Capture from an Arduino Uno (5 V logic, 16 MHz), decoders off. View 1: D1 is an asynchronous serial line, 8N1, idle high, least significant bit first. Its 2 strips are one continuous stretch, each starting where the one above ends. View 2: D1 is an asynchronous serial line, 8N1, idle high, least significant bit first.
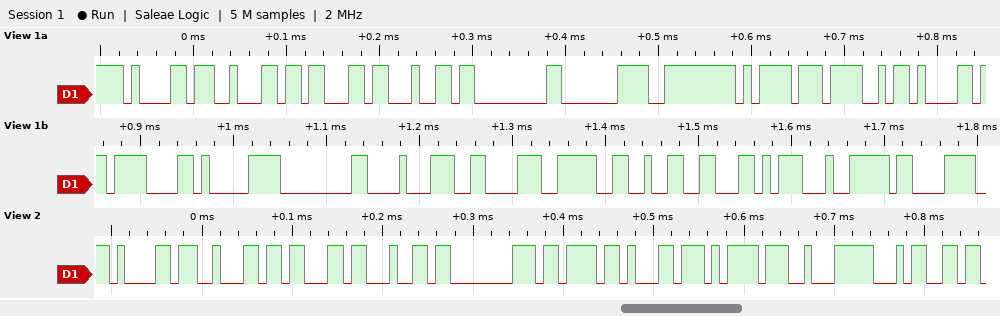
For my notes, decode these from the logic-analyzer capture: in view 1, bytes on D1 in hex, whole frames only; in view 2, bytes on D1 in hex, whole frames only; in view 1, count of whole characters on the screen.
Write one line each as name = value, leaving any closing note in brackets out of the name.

in view 1, bytes on D1 in hex, whole frames only = 0x61 0x62 0x63 0x64 0x00 0xC0 0xFE 0xBD 0x4F 0x61 0x0F 0xC1 0x00 0x88 0x86 0x3E 0x32 0xAC 0xE4 0xC3
in view 2, bytes on D1 in hex, whole frames only = 0x61 0x62 0x63 0x64 0x80 0x7B 0xB1 0xBD 0xE2 0x34
in view 1, count of whole characters on the screen = 20
